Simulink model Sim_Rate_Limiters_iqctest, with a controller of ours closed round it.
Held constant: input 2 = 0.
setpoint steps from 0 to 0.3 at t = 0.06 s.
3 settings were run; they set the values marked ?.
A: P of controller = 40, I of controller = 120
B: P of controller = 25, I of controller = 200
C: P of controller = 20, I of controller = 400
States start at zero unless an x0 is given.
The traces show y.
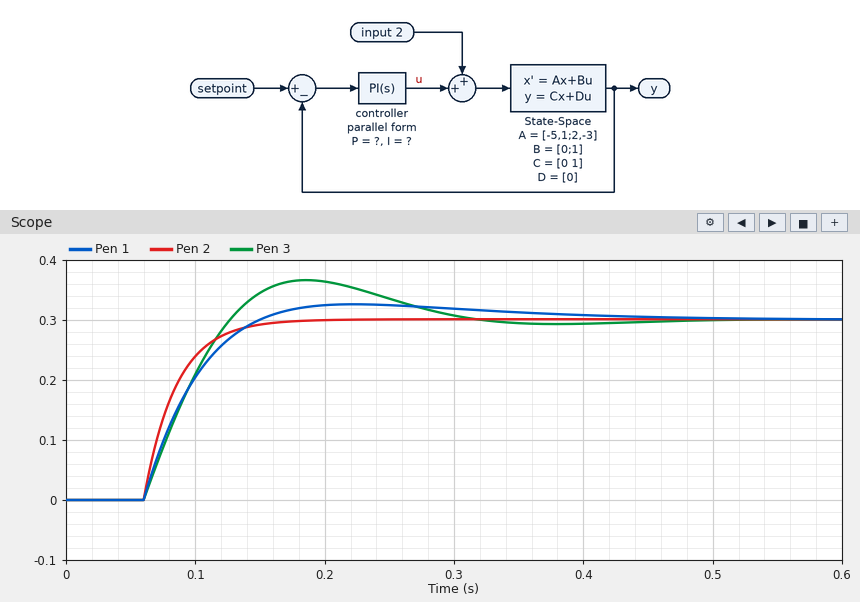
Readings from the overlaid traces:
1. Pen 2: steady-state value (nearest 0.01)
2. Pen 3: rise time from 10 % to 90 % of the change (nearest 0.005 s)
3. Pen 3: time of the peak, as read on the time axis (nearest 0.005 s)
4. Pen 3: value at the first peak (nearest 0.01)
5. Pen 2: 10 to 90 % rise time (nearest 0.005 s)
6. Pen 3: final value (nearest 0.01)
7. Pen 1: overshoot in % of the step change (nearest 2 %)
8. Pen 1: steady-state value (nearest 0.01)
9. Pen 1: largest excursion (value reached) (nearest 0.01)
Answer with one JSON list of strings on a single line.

["0.30", "0.050 s", "0.185 s", "0.37", "0.055 s", "0.30", "8 %", "0.30", "0.33"]
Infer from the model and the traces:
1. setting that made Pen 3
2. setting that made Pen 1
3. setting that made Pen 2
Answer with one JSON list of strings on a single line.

["C", "B", "A"]
